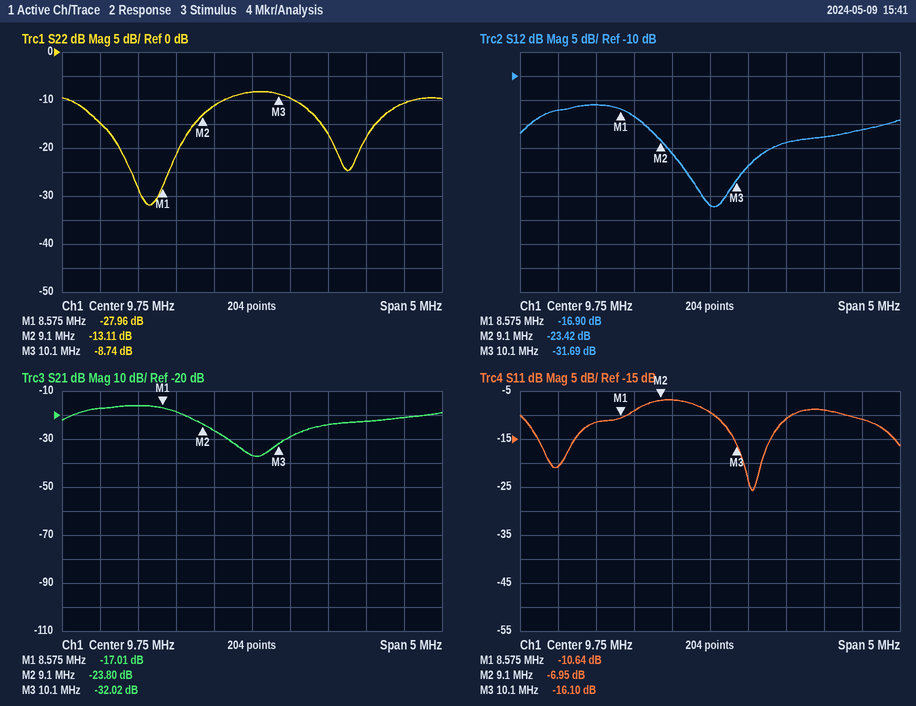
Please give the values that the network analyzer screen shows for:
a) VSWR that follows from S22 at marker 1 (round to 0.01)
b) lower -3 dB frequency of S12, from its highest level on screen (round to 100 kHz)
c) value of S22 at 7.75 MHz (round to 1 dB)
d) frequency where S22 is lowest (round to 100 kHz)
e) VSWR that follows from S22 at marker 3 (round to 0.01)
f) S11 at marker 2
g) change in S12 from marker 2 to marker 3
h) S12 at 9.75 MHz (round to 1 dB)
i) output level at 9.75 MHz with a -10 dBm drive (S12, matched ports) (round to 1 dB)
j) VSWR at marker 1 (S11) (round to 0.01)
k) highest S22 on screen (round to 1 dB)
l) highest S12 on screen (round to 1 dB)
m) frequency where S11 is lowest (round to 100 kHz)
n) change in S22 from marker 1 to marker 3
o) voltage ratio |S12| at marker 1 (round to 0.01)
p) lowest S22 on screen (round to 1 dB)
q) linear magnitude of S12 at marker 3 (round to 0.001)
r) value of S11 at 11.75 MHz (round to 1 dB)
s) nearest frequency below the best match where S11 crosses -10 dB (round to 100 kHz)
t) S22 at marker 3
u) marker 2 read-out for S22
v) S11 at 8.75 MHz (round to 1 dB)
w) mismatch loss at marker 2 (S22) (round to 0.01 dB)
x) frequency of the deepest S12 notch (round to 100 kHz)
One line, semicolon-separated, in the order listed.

1.08; 7.5 MHz; -15 dB; 8.4 MHz; 2.15; -6.95 dB; -8.27 dB; -37 dB; -47 dBm; 1.83; -8 dB; -16 dB; 10.3 MHz; 19.22 dB; 0.14; -32 dB; 0.026; -11 dB; 9.8 MHz; -8.74 dB; -13.11 dB; -9 dB; 0.22 dB; 9.8 MHz
